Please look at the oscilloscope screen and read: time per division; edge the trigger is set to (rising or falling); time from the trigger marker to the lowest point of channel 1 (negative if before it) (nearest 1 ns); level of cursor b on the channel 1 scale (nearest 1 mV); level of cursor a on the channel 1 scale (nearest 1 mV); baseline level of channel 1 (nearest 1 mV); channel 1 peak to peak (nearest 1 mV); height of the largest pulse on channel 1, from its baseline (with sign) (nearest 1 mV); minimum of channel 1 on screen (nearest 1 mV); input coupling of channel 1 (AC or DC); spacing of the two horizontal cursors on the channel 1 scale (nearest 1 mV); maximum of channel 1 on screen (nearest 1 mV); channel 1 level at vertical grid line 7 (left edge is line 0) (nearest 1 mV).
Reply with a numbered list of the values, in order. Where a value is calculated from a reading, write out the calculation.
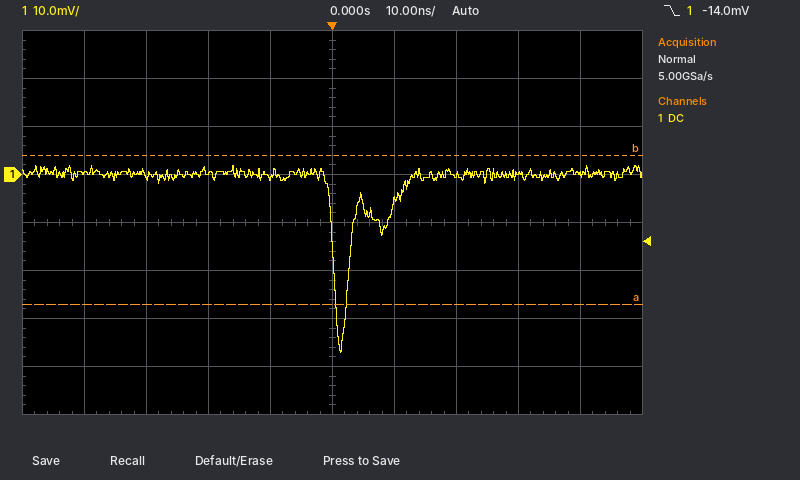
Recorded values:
1. 10 ns
2. falling
3. +1 ns
4. 4 mV
5. -27 mV
6. 0 mV
7. 2 mV − (-37 mV) = 39 mV
8. -37 mV − (0 mV) = -37 mV
9. -37 mV
10. DC
11. 31 mV
12. 2 mV
13. 0 mV
